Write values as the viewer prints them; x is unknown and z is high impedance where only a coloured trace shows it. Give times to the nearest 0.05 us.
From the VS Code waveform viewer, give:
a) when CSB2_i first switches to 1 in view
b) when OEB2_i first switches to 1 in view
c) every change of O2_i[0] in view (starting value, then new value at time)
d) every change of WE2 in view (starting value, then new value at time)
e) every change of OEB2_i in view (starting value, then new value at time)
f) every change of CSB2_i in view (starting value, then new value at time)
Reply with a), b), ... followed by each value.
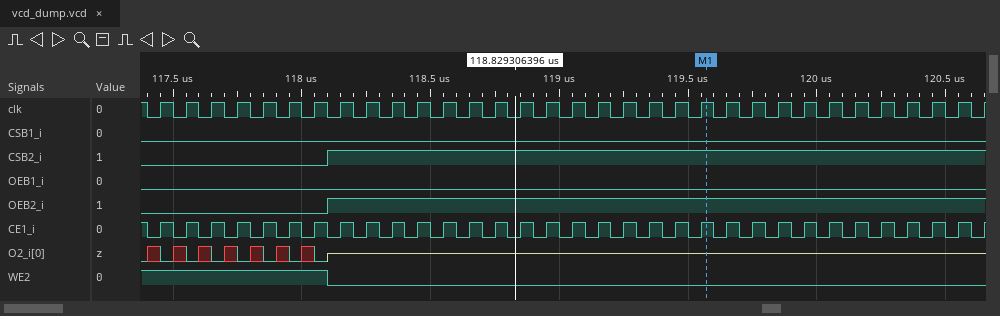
a) 118.1 us
b) 118.1 us
c) 0, x at 117.4 us, 0 at 117.45 us, x at 117.5 us, 0 at 117.55 us, x at 117.6 us, 0 at 117.65 us, x at 117.7 us, 0 at 117.75 us, x at 117.8 us, 0 at 117.85 us, x at 117.9 us, 0 at 117.95 us, x at 118 us, 0 at 118.05 us, z at 118.1 us
d) 1, 0 at 118.1 us
e) 0, 1 at 118.1 us
f) 0, 1 at 118.1 us
